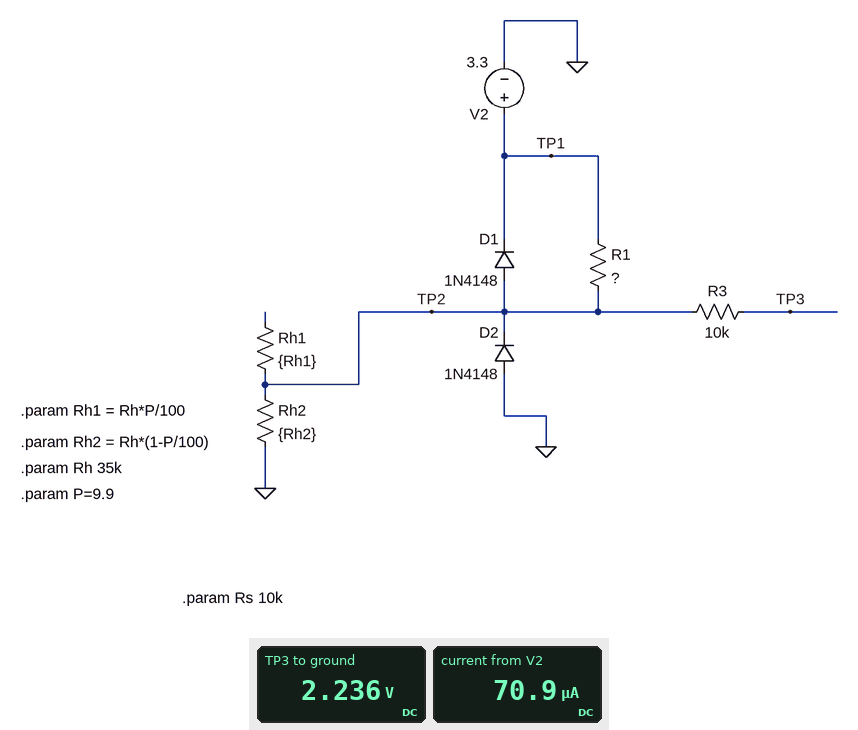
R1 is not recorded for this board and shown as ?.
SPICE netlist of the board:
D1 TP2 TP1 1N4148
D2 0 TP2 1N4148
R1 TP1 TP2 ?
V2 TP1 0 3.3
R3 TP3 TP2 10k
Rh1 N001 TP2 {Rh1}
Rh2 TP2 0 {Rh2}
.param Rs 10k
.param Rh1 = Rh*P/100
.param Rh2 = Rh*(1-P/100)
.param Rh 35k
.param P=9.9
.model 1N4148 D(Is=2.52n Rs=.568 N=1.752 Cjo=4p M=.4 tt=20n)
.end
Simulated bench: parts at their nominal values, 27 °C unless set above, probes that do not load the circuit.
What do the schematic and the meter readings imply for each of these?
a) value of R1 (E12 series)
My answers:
15 kΩ
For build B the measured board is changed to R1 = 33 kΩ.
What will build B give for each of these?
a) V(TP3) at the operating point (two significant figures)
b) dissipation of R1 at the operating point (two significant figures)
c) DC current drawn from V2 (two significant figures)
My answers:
1.6 V
86 µW
51 µA
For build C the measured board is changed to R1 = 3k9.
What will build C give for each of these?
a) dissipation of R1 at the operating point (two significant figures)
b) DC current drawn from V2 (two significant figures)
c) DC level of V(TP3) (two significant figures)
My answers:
34 µW
93 µA
2.9 V
